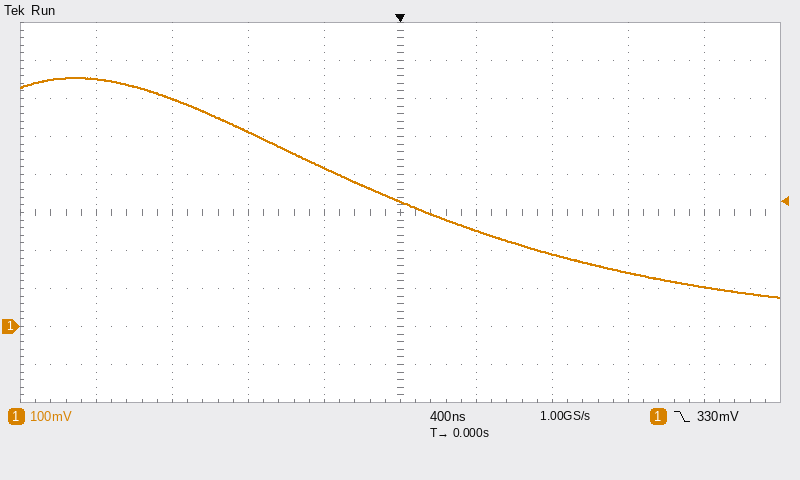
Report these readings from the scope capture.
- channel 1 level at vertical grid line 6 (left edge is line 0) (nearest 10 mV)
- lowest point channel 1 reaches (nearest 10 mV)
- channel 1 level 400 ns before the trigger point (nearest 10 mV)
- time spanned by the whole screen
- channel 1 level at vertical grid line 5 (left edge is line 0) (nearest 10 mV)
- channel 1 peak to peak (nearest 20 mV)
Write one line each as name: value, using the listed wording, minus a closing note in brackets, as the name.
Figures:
channel 1 level at vertical grid line 6 (left edge is line 0): 250 mV
lowest point channel 1 reaches: 80 mV
channel 1 level 400 ns before the trigger point: 420 mV
time spanned by the whole screen: 4 µs
channel 1 level at vertical grid line 5 (left edge is line 0): 330 mV
channel 1 peak to peak: 580 mV
